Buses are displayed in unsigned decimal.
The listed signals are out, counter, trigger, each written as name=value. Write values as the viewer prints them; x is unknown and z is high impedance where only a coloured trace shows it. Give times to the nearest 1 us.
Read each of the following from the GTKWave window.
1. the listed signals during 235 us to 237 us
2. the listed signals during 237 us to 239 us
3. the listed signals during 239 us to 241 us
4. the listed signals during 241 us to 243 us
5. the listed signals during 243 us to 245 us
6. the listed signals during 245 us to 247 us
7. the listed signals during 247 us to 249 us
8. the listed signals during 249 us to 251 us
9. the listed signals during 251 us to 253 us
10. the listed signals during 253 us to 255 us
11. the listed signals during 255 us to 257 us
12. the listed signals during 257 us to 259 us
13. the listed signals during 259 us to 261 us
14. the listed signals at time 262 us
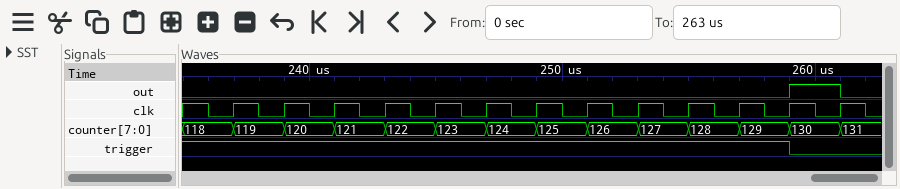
out=0, counter=118, trigger=1
out=0, counter=119, trigger=1
out=0, counter=120, trigger=1
out=0, counter=121, trigger=1
out=0, counter=122, trigger=1
out=0, counter=123, trigger=1
out=0, counter=124, trigger=1
out=0, counter=125, trigger=1
out=0, counter=126, trigger=1
out=0, counter=127, trigger=1
out=0, counter=128, trigger=1
out=0, counter=129, trigger=1
out=1, counter=130, trigger=0
out=0, counter=131, trigger=0
